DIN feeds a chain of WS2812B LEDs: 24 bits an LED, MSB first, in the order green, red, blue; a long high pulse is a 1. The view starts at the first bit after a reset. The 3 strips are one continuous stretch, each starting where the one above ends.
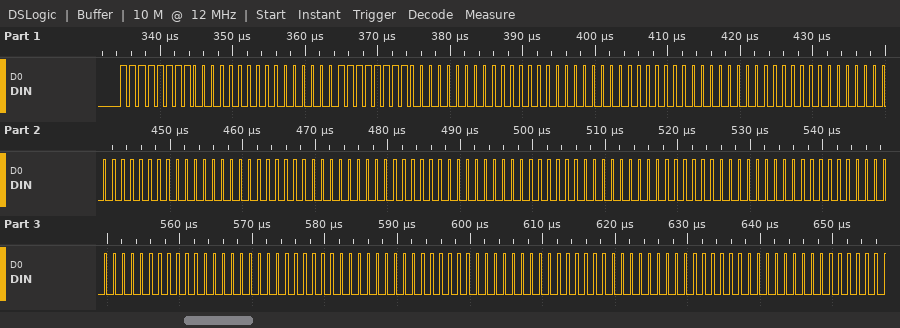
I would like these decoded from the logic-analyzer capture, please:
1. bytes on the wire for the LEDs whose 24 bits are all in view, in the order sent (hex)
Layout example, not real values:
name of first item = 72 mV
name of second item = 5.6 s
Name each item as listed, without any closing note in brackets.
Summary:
bytes on the wire for the LEDs whose 24 bits are all in view, in the order sent = FF 00 00 FF 00 00 00 00 00 00 00 00 00 00 00 00 00 00 00 00 00 00 00 00 00 00 00 00 00 00
